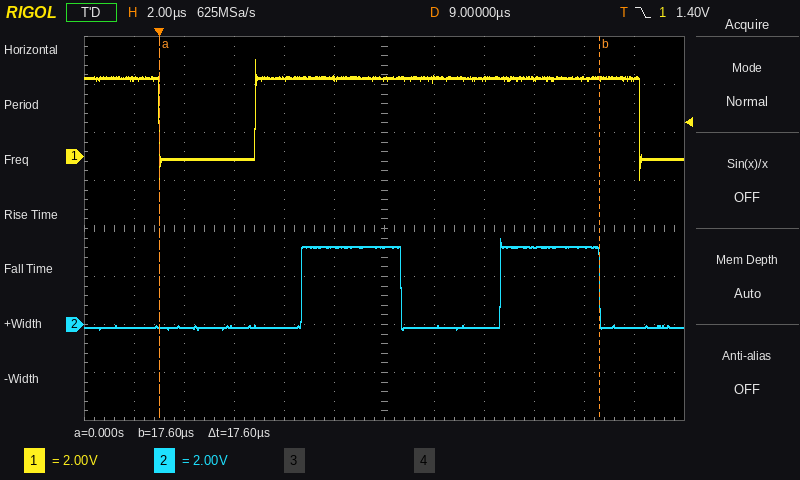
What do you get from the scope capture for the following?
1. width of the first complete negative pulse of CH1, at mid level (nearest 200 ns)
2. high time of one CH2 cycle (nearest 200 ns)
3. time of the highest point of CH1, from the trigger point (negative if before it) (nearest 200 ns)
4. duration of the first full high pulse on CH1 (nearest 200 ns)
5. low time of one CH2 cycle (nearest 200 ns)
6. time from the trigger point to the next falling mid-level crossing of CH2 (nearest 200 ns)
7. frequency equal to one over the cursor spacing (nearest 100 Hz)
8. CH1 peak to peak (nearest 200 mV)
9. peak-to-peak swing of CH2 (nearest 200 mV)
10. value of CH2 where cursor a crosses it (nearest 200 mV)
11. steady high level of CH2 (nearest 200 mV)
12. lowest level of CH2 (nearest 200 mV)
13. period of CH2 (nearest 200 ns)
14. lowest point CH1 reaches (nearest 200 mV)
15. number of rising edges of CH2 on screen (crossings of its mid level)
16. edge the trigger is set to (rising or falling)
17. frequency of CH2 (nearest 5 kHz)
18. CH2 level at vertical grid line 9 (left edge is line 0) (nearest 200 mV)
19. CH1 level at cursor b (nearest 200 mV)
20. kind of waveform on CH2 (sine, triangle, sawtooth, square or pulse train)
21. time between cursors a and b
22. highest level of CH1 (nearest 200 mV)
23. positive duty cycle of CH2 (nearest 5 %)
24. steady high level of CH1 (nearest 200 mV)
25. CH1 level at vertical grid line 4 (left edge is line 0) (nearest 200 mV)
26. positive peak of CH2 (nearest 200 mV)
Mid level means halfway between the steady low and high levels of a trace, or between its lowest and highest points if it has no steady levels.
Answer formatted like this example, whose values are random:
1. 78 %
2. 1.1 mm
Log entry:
1. 3.8 µs
2. 4.0 µs
3. +3.8 µs
4. 15.4 µs
5. 4.0 µs
6. 9.6 µs
7. 56.8 kHz
8. 5.0 V
9. 3.8 V
10. 0.0 V
11. 3.2 V
12. -200 mV
13. 8.0 µs
14. -1.0 V
15. 2
16. falling
17. 125 kHz
18. 3.2 V
19. 3.2 V
20. square
21. 17.6 µs
22. 4.0 V
23. 50 %
24. 3.2 V
25. 3.2 V
26. 3.6 V
